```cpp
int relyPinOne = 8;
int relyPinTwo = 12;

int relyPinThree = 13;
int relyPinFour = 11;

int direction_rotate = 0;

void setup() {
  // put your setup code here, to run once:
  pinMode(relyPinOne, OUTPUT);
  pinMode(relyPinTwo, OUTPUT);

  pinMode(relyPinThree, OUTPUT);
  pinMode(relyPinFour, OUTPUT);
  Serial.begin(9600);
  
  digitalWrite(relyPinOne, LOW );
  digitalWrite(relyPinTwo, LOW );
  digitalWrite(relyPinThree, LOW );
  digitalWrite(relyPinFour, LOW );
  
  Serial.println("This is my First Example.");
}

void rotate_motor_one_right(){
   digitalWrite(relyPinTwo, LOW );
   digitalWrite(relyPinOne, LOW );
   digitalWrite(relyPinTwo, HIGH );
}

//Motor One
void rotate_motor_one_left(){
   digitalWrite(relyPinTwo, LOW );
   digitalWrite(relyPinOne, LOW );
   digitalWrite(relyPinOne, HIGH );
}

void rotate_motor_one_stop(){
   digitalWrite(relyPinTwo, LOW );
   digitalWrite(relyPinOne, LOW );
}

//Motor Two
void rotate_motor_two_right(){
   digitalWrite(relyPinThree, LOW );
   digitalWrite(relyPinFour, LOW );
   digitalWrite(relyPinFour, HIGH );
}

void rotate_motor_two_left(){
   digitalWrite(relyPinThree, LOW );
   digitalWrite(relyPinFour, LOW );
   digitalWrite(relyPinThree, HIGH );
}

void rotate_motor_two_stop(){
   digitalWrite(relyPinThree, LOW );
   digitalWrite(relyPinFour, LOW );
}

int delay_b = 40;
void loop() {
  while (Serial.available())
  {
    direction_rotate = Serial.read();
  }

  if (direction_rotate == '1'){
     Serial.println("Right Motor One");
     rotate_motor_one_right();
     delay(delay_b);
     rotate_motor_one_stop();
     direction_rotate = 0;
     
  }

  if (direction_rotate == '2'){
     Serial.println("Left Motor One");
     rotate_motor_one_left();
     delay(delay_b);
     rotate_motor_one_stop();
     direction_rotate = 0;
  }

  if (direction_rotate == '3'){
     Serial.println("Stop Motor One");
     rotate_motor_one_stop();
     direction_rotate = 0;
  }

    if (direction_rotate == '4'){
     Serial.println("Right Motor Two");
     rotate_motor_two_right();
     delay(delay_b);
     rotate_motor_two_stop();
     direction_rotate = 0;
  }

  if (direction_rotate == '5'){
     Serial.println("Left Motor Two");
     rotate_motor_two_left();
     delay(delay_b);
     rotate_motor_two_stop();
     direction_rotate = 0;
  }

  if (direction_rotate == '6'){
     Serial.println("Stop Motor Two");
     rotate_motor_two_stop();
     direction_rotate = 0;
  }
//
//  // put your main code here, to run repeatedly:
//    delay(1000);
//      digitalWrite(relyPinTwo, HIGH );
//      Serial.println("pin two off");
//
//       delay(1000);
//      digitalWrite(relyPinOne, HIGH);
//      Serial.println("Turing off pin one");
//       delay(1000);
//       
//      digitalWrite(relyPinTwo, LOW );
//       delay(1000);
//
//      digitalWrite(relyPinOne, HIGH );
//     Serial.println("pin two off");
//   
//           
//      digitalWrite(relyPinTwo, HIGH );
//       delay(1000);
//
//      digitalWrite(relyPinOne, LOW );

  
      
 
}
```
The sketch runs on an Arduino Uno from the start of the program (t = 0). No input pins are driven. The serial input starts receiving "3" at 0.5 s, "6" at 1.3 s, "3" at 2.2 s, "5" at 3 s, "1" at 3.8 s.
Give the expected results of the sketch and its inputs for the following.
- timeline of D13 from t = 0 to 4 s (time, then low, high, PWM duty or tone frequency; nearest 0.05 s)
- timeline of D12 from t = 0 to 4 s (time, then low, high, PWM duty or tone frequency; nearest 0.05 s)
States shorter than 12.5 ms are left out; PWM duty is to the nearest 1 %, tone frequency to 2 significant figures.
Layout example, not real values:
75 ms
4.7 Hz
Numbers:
0 s low; 3 s high; 3.05 s low
0 s low; 3.8 s high; 3.85 s low
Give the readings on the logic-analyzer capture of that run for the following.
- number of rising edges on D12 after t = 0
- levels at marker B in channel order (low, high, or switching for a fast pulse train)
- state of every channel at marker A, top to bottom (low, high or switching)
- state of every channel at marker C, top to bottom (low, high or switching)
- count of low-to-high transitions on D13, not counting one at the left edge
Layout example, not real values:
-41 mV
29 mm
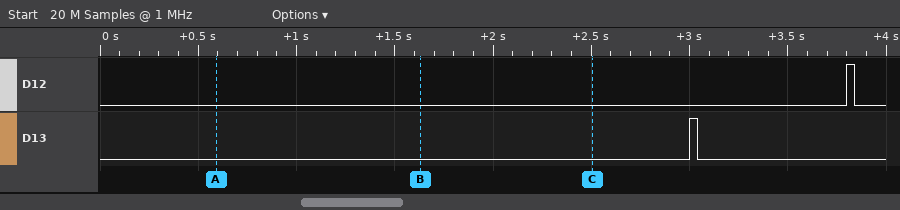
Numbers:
1
D12 low, D13 low
D12 low, D13 low
D12 low, D13 low
1
